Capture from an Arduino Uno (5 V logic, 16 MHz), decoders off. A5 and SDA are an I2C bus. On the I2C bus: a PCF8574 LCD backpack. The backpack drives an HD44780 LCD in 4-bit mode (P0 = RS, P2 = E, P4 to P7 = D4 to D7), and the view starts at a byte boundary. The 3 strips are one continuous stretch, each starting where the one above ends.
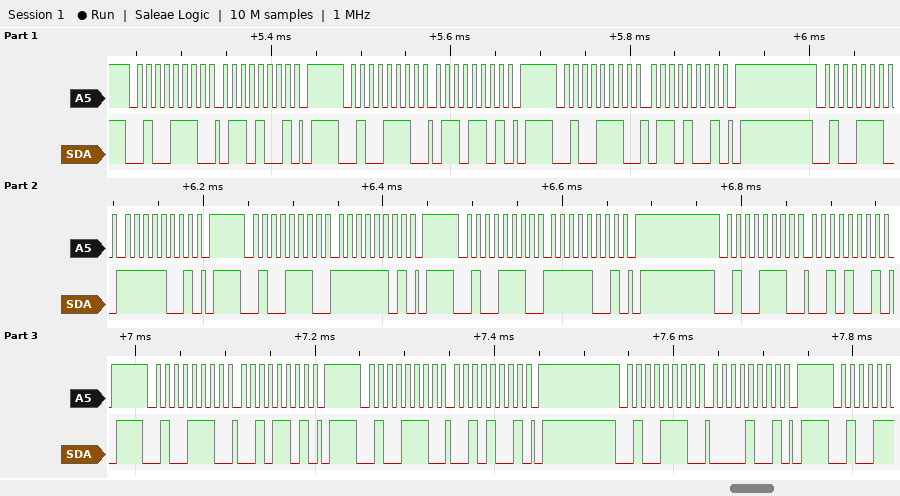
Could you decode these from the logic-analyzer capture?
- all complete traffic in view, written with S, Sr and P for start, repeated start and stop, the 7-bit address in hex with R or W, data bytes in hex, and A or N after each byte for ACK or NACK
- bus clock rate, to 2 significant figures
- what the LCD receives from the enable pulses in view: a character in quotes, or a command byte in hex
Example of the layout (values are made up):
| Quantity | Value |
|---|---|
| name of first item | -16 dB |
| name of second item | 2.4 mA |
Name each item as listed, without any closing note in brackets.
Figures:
| Quantity | Value |
|---|---|
| all complete traffic in view, written with S, Sr and P for start, repeated start and stop, the 7-bit address in hex with R or W, data bytes in hex, and A or N after each byte for ACK or NACK | S 27W A 69 A P S 27W A 6D A P S 27W A 69 A P S 27W A F9 A P S 27W A FD A P S 27W A F9 A P S 27W A 29 A P S 27W A 2D A P S 27W A 29 A P S 27W A 09 A P |
| bus clock rate, to 2 significant figures | 100 kHz |
| what the LCD receives from the enable pulses in view: a character in quotes, or a command byte in hex | 'o' |
